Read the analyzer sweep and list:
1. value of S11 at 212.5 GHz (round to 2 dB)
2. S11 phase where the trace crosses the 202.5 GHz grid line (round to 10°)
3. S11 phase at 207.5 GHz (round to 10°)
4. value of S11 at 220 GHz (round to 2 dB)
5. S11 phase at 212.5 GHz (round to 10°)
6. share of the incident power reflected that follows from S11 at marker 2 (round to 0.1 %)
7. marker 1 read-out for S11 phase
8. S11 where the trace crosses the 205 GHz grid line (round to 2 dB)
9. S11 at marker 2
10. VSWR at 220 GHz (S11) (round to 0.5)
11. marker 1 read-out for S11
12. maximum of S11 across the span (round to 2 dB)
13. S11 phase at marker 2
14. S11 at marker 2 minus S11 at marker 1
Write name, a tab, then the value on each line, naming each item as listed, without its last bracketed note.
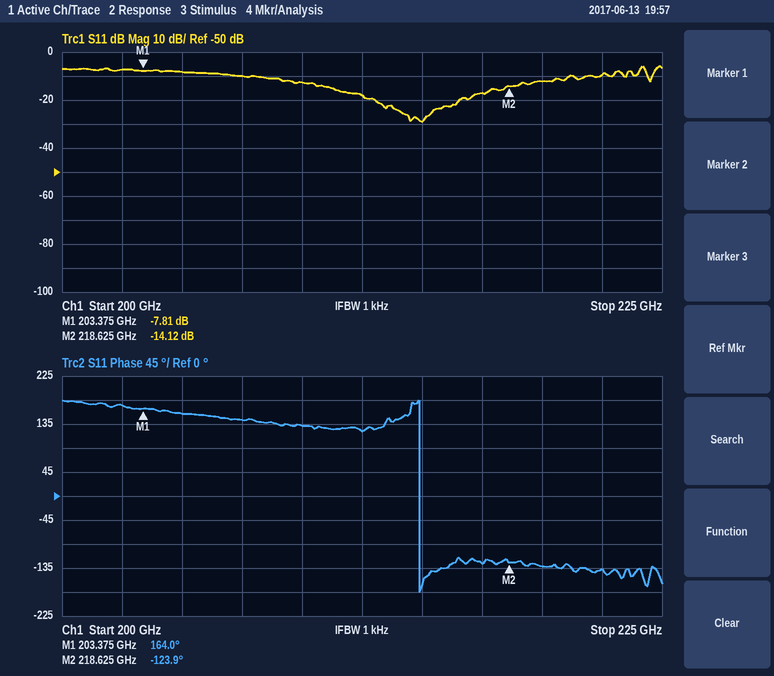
value of S11 at 212.5 GHz	-18 dB
S11 phase where the trace crosses the 202.5 GHz grid line	170°
S11 phase at 207.5 GHz	140°
value of S11 at 220 GHz	-12 dB
S11 phase at 212.5 GHz	120°
share of the incident power reflected that follows from S11 at marker 2	3.9 %
marker 1 read-out for S11 phase	164.0°
S11 where the trace crosses the 205 GHz grid line	-8 dB
S11 at marker 2	-14.12 dB
VSWR at 220 GHz (S11)	1.5
marker 1 read-out for S11	-7.81 dB
maximum of S11 across the span	-6 dB
S11 phase at marker 2	-123.9°
S11 at marker 2 minus S11 at marker 1	-6.31 dB
